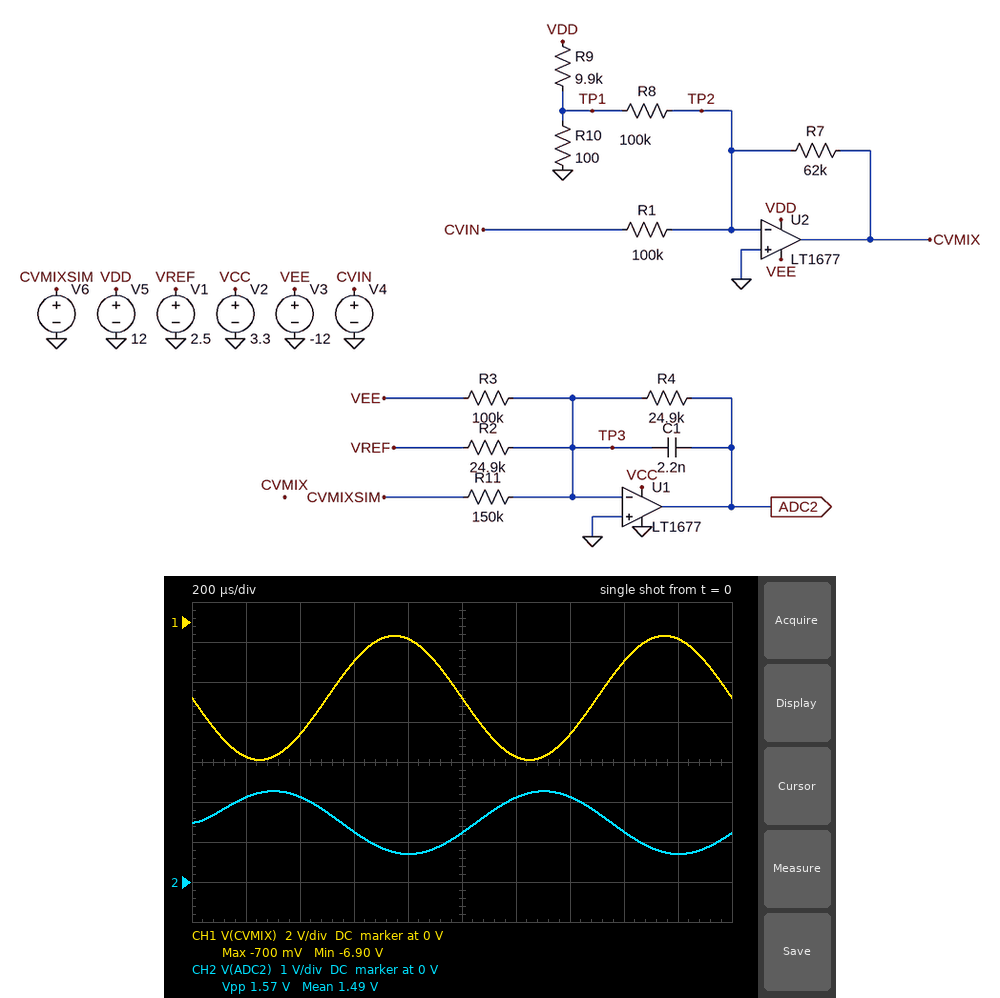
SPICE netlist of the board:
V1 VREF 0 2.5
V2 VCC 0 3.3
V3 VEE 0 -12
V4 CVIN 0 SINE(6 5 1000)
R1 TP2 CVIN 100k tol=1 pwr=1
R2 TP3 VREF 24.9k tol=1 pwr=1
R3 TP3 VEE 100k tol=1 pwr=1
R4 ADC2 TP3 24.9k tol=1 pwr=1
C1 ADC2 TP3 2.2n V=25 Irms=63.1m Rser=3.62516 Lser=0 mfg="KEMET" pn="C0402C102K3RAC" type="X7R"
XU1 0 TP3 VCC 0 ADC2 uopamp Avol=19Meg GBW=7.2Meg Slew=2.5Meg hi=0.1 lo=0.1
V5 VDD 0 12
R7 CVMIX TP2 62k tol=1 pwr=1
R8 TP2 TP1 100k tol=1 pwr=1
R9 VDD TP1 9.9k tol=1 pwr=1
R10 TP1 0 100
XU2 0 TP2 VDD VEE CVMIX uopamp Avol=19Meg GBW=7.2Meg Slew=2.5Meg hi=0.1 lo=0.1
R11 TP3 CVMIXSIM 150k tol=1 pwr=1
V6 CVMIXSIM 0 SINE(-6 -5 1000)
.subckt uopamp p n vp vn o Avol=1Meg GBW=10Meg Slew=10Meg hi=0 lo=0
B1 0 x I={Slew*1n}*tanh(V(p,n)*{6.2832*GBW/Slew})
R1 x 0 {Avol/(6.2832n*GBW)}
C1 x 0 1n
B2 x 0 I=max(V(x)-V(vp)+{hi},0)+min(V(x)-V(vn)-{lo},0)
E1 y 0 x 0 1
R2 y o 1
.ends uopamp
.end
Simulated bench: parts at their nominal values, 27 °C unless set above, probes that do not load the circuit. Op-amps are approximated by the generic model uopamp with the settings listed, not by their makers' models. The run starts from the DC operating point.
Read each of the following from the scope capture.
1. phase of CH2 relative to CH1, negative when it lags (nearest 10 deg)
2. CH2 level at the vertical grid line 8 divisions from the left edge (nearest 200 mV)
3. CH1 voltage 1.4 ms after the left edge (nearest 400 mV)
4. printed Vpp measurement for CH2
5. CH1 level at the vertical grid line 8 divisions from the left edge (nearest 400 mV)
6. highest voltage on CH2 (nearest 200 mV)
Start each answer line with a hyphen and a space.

- 160 deg
- 1.2 V
- -5.6 V
- 1.57 V
- -2.0 V
- 2.2 V
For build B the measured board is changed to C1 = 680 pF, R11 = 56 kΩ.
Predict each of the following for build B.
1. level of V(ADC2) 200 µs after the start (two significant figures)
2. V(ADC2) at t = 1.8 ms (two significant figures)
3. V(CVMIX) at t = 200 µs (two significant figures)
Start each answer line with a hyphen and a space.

- 3.2 V
- 990 mV
- -6.7 V
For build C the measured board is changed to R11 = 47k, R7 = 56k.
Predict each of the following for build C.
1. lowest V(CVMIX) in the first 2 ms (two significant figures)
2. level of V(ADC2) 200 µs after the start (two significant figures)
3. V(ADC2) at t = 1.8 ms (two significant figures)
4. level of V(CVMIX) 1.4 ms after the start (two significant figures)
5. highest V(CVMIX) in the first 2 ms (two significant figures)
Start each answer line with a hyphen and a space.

- -6.2 V
- 3.2 V
- 1.2 V
- -5.1 V
- -630 mV
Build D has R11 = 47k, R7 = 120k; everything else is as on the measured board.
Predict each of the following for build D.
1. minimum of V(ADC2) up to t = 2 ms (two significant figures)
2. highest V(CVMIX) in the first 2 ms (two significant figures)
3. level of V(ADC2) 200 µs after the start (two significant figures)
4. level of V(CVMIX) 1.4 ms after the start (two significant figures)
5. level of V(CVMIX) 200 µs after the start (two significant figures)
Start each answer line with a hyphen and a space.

- 1.2 V
- -1.3 V
- 3.2 V
- -11 V
- -12 V
